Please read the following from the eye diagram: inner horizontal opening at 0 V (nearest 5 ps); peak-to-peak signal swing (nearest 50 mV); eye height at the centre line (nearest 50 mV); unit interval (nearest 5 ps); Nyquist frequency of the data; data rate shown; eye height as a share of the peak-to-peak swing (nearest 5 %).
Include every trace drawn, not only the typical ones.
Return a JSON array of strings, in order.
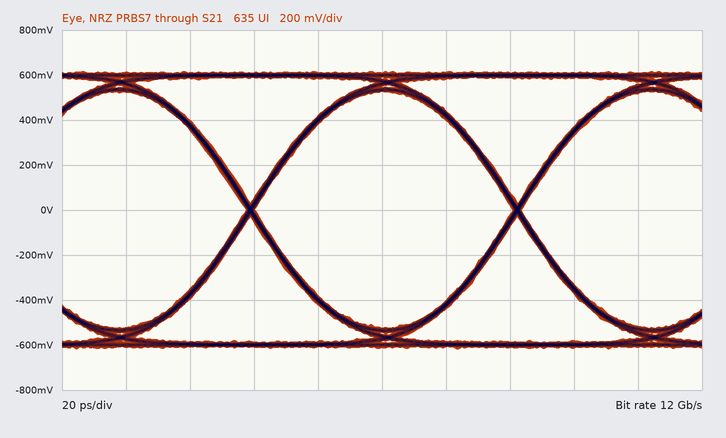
["80 ps", "1.25 V", "1.05 V", "85 ps", "6 GHz", "12 Gb/s", "85 %"]
